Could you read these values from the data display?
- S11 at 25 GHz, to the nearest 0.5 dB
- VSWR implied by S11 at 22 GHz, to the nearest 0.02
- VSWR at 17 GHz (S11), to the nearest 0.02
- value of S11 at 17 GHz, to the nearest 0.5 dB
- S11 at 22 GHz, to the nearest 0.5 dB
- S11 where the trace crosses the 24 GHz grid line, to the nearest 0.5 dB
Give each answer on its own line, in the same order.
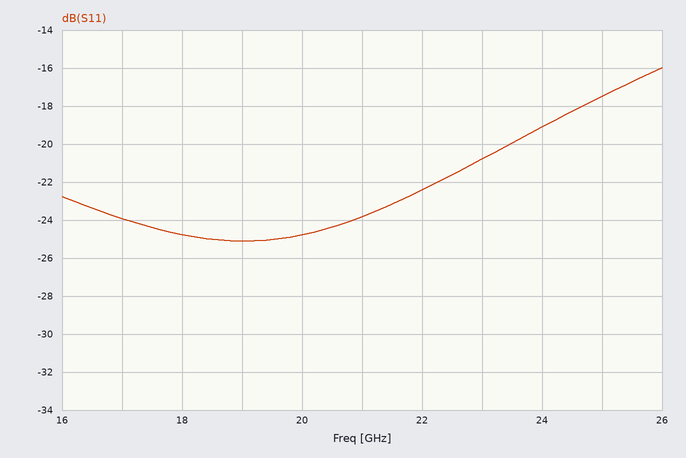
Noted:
-17.5 dB
1.16
1.14
-24.0 dB
-22.5 dB
-19.0 dB
